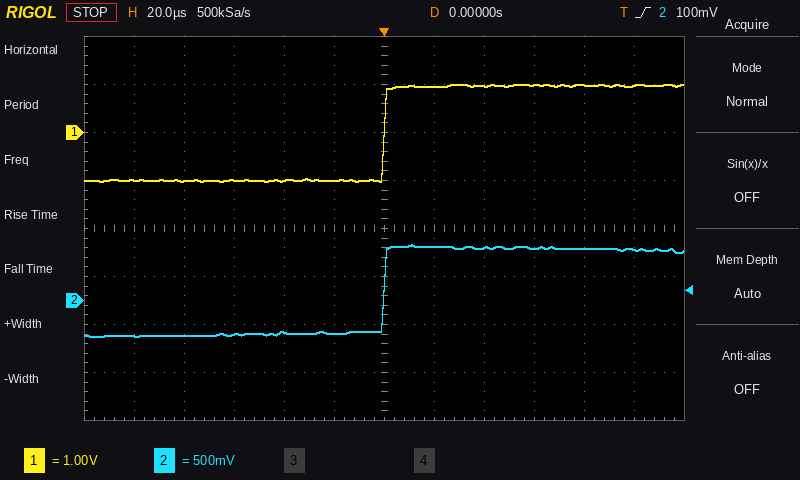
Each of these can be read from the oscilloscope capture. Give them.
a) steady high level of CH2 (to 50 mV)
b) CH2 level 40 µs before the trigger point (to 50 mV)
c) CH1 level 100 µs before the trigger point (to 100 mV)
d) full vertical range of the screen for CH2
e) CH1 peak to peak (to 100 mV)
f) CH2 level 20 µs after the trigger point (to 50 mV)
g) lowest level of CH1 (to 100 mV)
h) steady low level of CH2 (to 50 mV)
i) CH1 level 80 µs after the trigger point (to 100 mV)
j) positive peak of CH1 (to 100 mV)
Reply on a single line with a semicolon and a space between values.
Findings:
550 mV; -350 mV; -1.0 V; 4 V; 2.0 V; 550 mV; -1.0 V; -350 mV; 1.0 V; 1.0 V
